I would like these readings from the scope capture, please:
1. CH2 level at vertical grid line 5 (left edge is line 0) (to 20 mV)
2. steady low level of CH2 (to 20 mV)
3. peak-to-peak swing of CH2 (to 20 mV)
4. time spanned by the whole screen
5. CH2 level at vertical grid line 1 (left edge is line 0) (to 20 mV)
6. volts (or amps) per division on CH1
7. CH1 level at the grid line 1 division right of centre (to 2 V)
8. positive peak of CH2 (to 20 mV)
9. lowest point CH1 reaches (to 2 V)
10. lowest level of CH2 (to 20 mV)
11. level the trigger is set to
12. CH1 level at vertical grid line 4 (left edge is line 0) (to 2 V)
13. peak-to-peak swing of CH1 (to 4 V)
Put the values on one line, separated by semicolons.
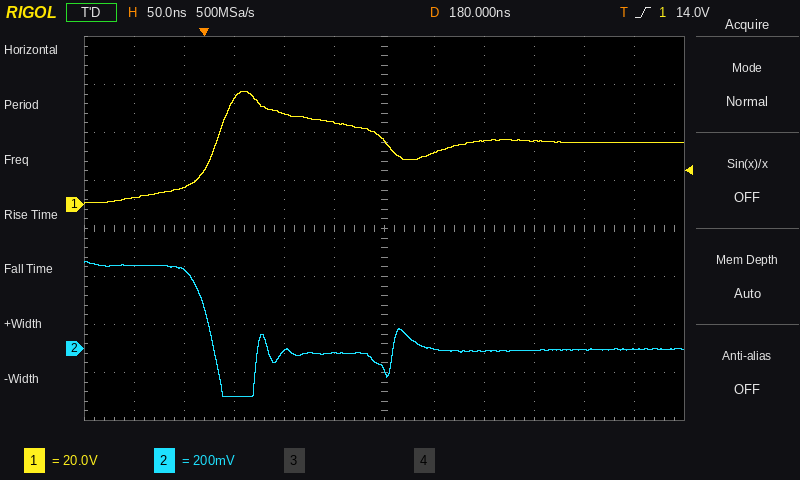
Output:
-20 mV; 0 mV; 560 mV; 600 ns; 340 mV; 20 V; 22 V; 360 mV; 0 V; -200 mV; 14.0 V; 38 V; 48 V
